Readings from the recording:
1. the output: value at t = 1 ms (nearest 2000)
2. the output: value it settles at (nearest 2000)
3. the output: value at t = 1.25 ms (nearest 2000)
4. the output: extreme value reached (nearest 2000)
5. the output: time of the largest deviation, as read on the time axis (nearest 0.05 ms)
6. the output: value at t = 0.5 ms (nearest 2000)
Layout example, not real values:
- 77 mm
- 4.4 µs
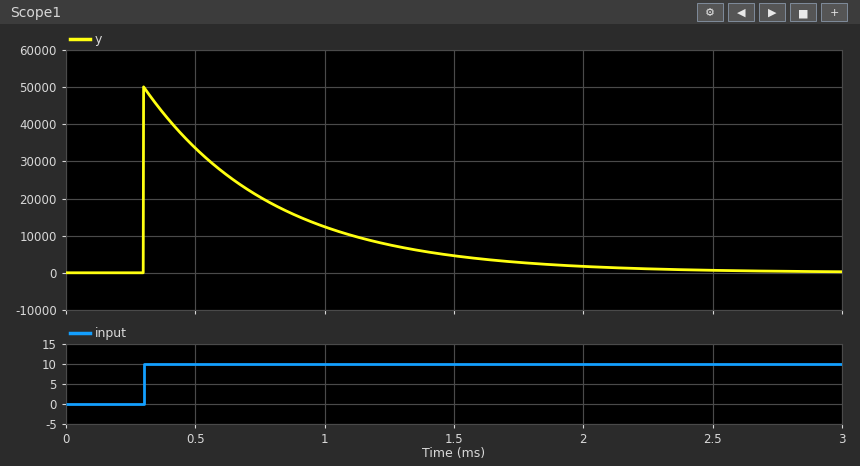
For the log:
- 12000
- 0
- 8000
- 50000
- 0.30 ms
- 34000
